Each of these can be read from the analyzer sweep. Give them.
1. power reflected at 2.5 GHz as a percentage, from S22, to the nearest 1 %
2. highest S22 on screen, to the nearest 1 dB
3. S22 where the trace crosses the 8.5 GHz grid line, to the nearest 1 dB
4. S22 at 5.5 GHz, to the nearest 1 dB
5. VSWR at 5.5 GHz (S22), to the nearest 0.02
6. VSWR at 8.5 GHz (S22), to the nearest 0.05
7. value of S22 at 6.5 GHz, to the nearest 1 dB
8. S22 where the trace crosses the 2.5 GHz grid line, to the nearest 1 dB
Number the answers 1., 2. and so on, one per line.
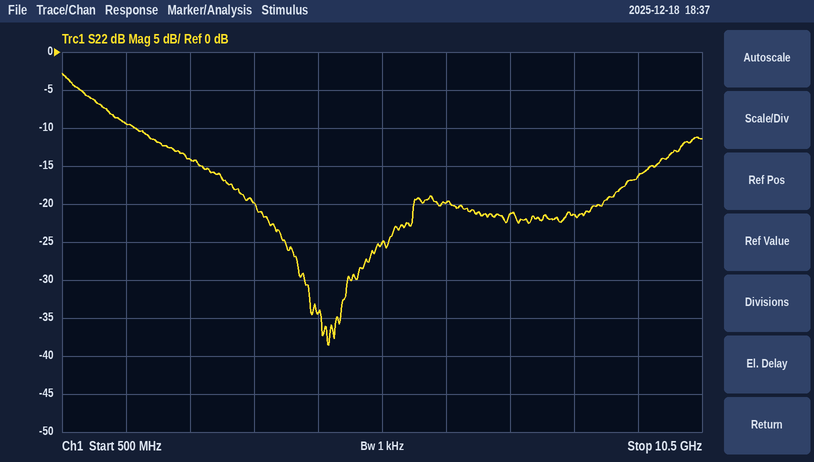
1. 4 %
2. -3 dB
3. -21 dB
4. -25 dB
5. 1.12
6. 1.20
7. -20 dB
8. -14 dB
